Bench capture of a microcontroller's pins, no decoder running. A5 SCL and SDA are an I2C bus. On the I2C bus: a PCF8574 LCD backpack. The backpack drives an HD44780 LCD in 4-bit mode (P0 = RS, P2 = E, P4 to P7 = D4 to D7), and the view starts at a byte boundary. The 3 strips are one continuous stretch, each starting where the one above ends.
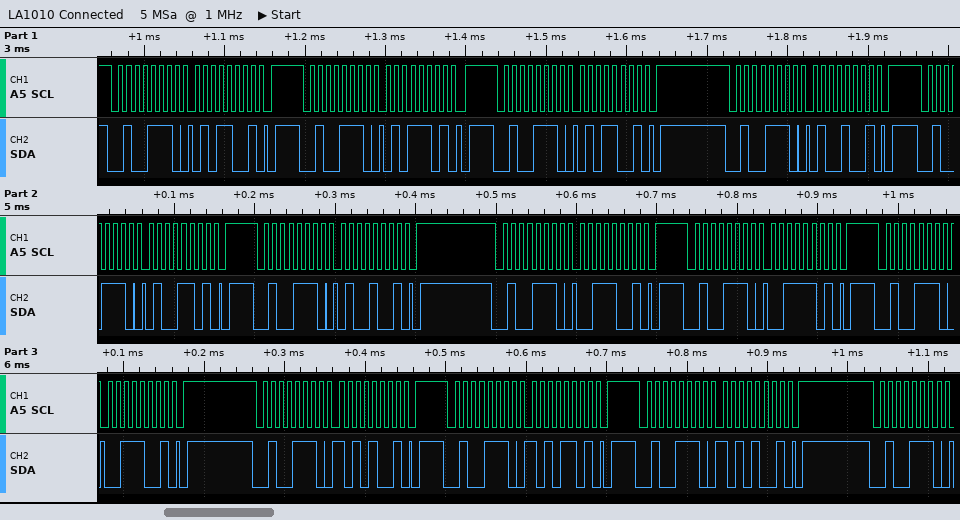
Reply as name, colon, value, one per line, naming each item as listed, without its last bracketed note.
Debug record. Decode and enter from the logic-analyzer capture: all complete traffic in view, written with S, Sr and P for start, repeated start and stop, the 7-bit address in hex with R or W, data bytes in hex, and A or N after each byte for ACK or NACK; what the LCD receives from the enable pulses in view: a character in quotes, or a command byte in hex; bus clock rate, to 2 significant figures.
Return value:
all complete traffic in view, written with S, Sr and P for start, repeated start and stop, the 7-bit address in hex with R or W, data bytes in hex, and A or N after each byte for ACK or NACK: S 27W A 59 A P S 27W A 5D A P S 27W A 59 A P S 27W A 49 A P S 27W A 4D A P S 27W A 49 A P S 27W A 39 A P S 27W A 3D A P S 27W A 39 A P S 27W A A9 A P S 27W A AD A P S 27W A A9 A P S 27W A
what the LCD receives from the enable pulses in view: a character in quotes, or a command byte in hex: 'T' ':'
bus clock rate, to 2 significant figures: 100 kHz
